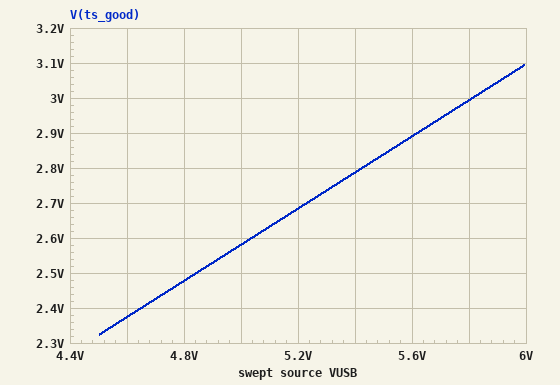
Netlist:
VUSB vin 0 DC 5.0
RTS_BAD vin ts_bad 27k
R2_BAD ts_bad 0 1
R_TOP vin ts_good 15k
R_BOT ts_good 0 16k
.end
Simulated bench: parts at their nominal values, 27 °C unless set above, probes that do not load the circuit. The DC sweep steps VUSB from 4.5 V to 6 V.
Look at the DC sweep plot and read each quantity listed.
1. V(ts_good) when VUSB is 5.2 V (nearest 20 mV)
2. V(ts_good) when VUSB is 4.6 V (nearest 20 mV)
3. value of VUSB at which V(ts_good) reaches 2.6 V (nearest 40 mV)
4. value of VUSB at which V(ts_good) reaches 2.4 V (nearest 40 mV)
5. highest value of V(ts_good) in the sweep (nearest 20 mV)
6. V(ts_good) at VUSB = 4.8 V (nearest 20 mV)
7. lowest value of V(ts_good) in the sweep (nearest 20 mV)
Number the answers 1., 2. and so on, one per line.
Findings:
1. 2.68 V
2. 2.38 V
3. 5.04 V
4. 4.64 V
5. 3.10 V
6. 2.48 V
7. 2.32 V
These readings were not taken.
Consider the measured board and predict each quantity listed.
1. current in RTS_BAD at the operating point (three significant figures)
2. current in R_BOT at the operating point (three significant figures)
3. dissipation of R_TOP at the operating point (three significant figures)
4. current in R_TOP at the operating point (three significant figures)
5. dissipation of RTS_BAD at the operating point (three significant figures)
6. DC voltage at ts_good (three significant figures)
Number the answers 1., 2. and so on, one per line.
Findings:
1. 185 µA
2. 161 µA
3. 390 µW
4. 161 µA
5. 926 µW
6. 2.58 V
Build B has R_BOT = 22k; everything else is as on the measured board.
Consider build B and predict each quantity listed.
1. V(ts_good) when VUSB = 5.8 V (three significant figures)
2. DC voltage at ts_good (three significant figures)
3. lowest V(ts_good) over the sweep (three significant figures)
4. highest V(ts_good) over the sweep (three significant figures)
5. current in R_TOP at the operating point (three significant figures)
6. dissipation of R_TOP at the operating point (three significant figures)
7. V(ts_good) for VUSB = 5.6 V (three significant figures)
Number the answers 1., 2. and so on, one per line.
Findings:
1. 3.45 V
2. 2.97 V
3. 2.68 V
4. 3.57 V
5. 135 µA
6. 274 µW
7. 3.33 V
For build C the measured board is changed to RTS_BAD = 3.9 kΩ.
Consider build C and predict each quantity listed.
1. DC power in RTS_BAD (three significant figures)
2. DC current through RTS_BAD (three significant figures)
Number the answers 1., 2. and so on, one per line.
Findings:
1. 6.41 mW
2. 1.28 mA
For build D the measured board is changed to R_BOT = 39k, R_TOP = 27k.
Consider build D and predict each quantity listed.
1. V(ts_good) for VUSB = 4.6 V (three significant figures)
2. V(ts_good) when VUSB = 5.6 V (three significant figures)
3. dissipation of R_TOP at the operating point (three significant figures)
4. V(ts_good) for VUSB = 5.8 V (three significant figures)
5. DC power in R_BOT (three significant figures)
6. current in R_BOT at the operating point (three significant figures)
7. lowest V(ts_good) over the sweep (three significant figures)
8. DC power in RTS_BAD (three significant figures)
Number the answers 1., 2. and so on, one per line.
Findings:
1. 2.72 V
2. 3.31 V
3. 155 µW
4. 3.43 V
5. 224 µW
6. 75.8 µA
7. 2.66 V
8. 926 µW
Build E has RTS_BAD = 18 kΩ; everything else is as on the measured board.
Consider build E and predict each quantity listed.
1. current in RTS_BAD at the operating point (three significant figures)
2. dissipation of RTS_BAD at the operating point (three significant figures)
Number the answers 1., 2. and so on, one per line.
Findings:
1. 278 µA
2. 1.39 mW
